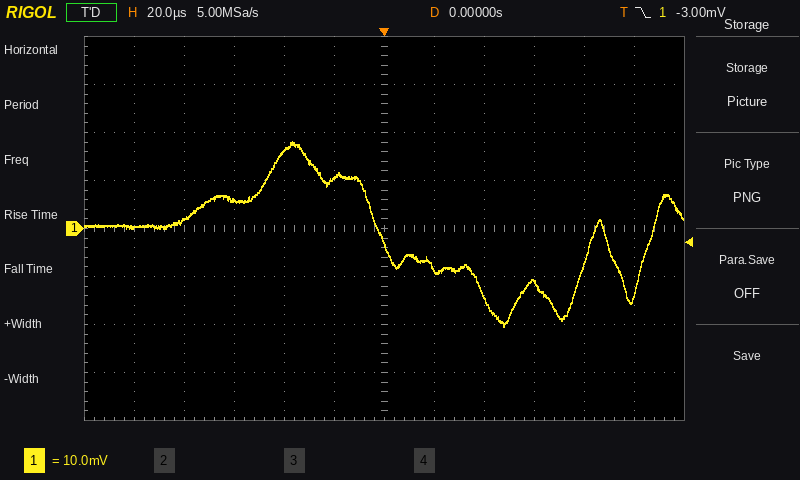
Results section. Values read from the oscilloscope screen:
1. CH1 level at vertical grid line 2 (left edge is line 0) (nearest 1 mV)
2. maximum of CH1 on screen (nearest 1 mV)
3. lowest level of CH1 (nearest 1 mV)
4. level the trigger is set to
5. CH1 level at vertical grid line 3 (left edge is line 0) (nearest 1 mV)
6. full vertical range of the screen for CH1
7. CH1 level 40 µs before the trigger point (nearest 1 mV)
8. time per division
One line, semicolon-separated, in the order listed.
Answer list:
2 mV; 18 mV; -20 mV; -3.00 mV; 6 mV; 80 mV; 16 mV; 20 µs
